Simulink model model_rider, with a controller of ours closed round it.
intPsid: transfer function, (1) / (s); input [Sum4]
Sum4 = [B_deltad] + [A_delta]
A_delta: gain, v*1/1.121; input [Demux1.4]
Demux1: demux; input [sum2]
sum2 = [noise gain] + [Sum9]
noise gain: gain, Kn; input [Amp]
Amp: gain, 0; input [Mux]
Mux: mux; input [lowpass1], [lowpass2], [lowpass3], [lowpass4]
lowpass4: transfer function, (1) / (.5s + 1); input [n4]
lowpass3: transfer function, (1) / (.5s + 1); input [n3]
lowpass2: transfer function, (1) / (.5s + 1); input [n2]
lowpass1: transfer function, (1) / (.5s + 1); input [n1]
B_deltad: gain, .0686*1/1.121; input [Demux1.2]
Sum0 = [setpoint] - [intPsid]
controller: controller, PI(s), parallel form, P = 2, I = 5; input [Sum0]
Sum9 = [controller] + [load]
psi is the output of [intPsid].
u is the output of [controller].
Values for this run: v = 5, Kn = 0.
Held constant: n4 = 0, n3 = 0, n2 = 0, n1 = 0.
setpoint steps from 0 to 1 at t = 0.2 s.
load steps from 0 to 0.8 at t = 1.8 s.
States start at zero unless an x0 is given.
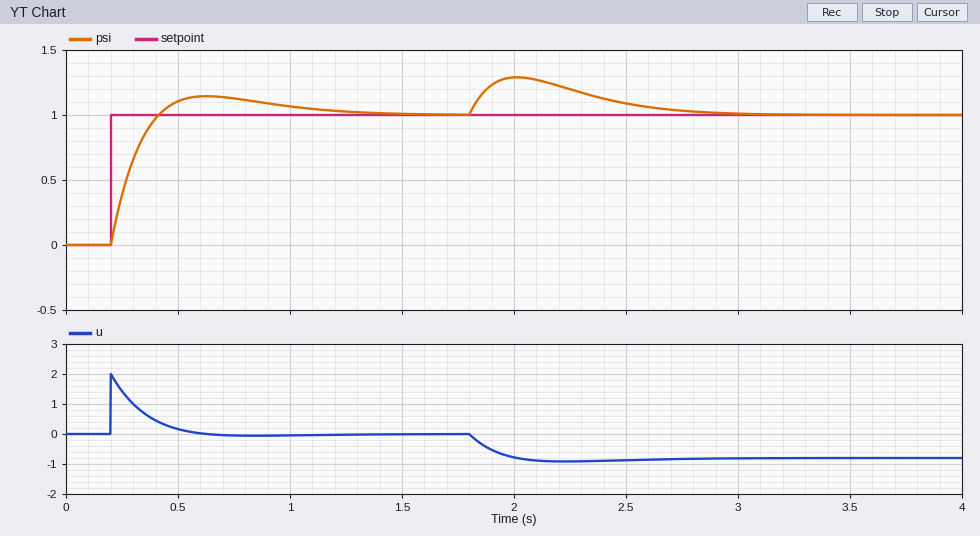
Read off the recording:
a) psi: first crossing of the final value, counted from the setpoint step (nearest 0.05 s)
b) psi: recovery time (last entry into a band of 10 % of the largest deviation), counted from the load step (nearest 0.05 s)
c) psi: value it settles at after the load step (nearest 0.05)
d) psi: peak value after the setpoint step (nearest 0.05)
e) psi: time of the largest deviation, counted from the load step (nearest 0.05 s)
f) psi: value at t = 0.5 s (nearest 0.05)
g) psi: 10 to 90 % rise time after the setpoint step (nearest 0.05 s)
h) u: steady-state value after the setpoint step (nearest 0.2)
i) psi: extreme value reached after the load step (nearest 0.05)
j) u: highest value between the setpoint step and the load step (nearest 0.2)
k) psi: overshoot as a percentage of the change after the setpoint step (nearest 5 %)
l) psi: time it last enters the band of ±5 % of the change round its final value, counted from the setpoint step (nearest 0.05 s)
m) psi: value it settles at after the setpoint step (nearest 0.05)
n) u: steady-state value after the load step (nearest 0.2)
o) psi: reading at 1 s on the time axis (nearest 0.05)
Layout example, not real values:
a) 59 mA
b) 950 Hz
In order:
a) 0.20 s
b) 1.00 s
c) 1.00
d) 1.15
e) 0.20 s
f) 1.10
g) 0.15 s
h) 0.0
i) 1.30
j) 2.0
k) 15 %
l) 0.90 s
m) 1.00
n) -0.8
o) 1.05
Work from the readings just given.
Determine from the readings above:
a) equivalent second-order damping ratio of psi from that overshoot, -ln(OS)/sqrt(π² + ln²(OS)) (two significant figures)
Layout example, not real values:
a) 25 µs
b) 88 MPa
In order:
a) 0.52
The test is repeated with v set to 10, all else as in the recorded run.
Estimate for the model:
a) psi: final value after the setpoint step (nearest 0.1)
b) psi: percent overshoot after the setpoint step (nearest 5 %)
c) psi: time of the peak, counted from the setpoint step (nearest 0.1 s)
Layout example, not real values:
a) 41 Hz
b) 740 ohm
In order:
a) 1.0
b) 10 %
c) 0.3 s
